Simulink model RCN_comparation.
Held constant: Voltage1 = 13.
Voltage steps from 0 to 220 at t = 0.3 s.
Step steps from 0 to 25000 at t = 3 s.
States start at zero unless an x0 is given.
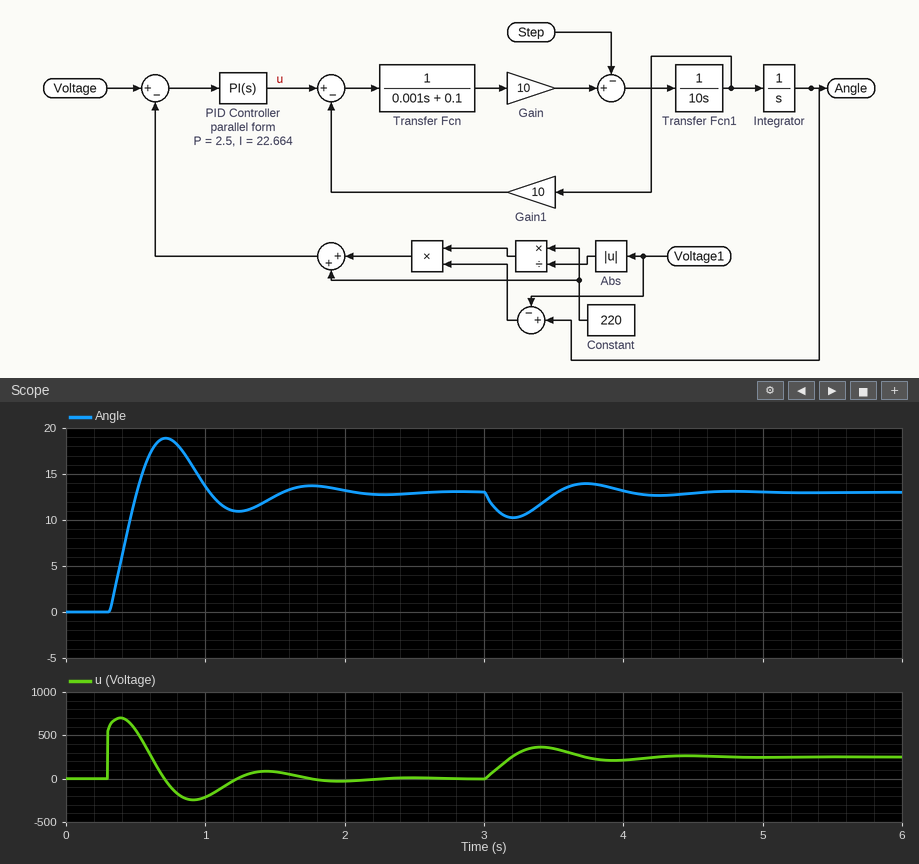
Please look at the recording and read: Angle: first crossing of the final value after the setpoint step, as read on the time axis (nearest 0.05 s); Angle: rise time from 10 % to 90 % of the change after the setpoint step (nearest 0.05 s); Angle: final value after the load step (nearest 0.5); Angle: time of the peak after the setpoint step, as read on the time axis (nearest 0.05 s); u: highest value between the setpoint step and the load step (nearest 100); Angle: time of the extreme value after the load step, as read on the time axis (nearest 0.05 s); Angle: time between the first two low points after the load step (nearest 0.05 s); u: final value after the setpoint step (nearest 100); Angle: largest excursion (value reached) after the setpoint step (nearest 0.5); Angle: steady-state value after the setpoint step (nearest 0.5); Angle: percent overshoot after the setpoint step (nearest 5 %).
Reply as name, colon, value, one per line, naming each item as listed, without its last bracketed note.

Angle: first crossing of the final value after the setpoint step, as read on the time axis: 0.50 s
Angle: rise time from 10 % to 90 % of the change after the setpoint step: 0.15 s
Angle: final value after the load step: 13.0
Angle: time of the peak after the setpoint step, as read on the time axis: 0.70 s
u: highest value between the setpoint step and the load step: 700
Angle: time of the extreme value after the load step, as read on the time axis: 3.20 s
Angle: time between the first two low points after the load step: 1.05 s
u: final value after the setpoint step: 0
Angle: largest excursion (value reached) after the setpoint step: 19.0
Angle: steady-state value after the setpoint step: 13.0
Angle: percent overshoot after the setpoint step: 45 %
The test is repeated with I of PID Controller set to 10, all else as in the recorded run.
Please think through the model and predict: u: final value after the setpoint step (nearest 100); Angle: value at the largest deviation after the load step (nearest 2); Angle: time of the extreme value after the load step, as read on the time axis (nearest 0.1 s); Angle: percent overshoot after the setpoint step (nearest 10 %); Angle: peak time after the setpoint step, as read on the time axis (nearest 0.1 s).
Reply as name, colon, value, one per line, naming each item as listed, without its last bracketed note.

u: final value after the setpoint step: 0
Angle: value at the largest deviation after the load step: 10
Angle: time of the extreme value after the load step, as read on the time axis: 3.3 s
Angle: percent overshoot after the setpoint step: 30 %
Angle: peak time after the setpoint step, as read on the time axis: 0.9 s
